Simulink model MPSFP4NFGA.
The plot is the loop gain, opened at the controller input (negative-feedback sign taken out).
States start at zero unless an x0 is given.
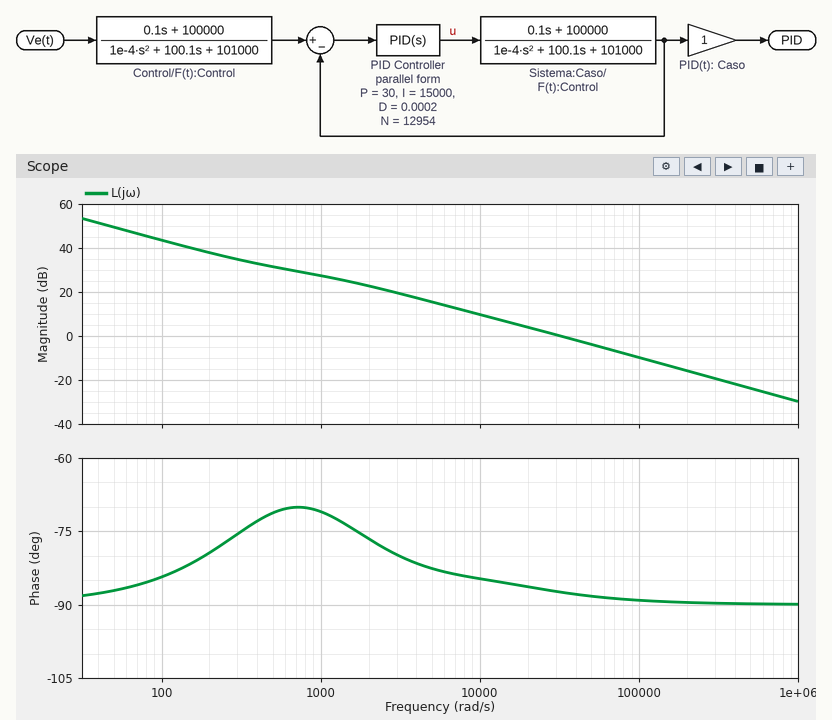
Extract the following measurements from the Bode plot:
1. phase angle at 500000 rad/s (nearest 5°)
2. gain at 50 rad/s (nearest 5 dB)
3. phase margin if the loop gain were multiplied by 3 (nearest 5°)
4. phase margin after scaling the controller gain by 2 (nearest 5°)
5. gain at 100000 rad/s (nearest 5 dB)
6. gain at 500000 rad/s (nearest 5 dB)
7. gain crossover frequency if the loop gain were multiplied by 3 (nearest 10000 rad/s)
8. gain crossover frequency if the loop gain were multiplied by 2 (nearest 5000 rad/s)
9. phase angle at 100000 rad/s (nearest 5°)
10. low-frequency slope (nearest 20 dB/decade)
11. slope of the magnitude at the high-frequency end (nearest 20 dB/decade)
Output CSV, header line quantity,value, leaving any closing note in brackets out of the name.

quantity,value
phase angle at 500000 rad/s,-90°
gain at 50 rad/s,50 dB
phase margin if the loop gain were multiplied by 3,90°
phase margin after scaling the controller gain by 2,90°
gain at 100000 rad/s,-10 dB
gain at 500000 rad/s,-25 dB
gain crossover frequency if the loop gain were multiplied by 3,100000 rad/s
gain crossover frequency if the loop gain were multiplied by 2,65000 rad/s
phase angle at 100000 rad/s,-90°
low-frequency slope,-20 dB/decade
slope of the magnitude at the high-frequency end,-20 dB/decade
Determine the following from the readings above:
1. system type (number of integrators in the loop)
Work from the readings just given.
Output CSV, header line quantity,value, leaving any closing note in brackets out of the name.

quantity,value
system type,1
